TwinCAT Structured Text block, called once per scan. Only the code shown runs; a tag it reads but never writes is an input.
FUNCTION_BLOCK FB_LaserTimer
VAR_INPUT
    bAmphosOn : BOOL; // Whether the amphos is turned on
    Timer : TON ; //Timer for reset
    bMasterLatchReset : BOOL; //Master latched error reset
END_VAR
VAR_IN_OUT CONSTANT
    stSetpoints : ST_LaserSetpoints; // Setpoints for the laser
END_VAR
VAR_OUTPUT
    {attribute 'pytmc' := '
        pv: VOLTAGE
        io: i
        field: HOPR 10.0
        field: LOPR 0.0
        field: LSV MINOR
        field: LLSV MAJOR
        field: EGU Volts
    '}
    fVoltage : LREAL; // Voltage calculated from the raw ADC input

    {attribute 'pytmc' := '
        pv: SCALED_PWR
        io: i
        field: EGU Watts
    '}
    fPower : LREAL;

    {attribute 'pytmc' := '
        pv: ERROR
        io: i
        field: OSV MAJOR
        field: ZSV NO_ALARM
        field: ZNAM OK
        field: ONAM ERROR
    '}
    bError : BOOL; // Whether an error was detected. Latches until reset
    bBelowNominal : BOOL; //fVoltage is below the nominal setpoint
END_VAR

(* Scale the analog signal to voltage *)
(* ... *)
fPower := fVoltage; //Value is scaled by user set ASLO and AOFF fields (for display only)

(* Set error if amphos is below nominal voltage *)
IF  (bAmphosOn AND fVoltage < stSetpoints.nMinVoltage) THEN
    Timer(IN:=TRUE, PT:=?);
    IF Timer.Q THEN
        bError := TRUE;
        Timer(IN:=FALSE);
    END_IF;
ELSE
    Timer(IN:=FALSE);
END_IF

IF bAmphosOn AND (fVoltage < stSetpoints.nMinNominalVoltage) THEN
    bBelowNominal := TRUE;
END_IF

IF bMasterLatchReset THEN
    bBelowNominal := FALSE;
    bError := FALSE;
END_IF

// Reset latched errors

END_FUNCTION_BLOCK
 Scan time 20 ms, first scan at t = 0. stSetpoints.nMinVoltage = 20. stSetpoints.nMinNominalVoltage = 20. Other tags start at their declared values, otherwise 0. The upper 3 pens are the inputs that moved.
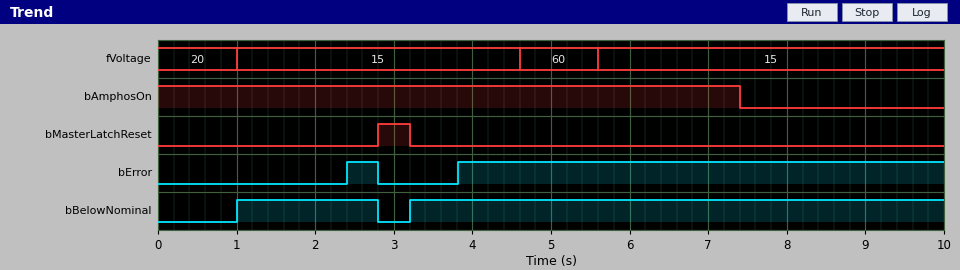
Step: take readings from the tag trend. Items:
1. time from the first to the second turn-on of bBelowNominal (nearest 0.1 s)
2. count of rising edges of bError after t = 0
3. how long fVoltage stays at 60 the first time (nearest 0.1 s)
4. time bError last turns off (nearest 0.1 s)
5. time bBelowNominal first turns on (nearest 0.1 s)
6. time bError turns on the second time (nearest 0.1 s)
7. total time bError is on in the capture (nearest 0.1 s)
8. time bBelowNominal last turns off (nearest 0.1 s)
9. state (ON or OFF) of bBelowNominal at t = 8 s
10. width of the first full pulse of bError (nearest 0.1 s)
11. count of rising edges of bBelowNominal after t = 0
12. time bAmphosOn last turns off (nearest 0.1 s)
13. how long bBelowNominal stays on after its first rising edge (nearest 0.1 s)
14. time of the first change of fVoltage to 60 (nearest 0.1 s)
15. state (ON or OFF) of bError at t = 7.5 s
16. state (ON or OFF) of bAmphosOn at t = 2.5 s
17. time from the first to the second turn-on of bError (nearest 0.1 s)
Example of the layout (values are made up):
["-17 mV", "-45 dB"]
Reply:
["2.2 s", "2", "1.0 s", "2.8 s", "1.0 s", "3.8 s", "6.6 s", "2.8 s", "ON", "0.4 s", "2", "7.4 s", "1.8 s", "4.6 s", "ON", "ON", "1.4 s"]
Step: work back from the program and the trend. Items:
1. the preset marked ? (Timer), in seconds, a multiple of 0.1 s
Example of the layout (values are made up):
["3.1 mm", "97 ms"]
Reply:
["1.4 s"]
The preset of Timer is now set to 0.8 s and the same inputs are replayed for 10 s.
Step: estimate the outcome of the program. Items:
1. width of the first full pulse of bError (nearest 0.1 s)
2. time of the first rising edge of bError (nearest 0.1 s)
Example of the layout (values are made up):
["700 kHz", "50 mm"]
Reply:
["1.0 s", "1.8 s"]
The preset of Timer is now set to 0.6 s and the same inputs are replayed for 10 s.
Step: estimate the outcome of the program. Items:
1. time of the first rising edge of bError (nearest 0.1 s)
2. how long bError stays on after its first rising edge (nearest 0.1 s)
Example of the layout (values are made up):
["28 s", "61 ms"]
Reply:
["1.6 s", "1.2 s"]
